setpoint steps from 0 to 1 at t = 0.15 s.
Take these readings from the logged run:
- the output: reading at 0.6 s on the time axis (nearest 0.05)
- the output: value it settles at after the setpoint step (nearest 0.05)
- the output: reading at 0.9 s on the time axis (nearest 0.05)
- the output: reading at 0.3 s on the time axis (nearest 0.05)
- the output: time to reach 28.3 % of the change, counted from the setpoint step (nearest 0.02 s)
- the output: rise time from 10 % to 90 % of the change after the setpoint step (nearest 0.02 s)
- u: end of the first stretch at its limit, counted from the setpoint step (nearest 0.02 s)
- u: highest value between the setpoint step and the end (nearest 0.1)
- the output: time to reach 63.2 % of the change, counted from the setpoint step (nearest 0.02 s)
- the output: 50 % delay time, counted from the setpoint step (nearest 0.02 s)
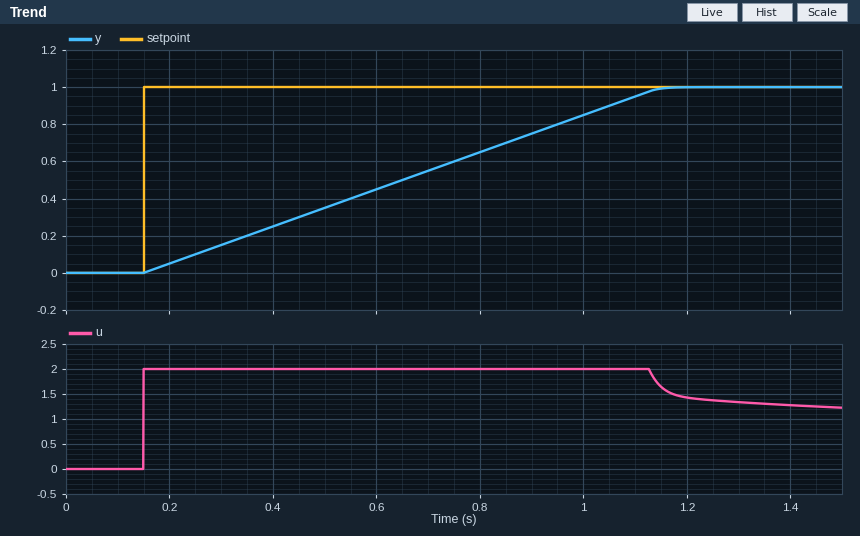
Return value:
0.45
1.00
0.75
0.15
0.28 s
0.80 s
0.98 s
2.0
0.64 s
0.50 s
